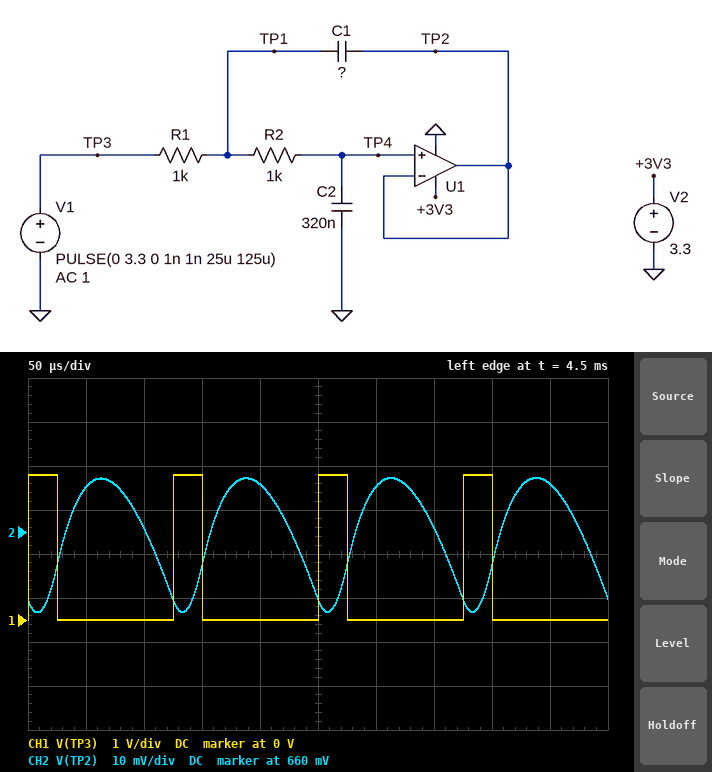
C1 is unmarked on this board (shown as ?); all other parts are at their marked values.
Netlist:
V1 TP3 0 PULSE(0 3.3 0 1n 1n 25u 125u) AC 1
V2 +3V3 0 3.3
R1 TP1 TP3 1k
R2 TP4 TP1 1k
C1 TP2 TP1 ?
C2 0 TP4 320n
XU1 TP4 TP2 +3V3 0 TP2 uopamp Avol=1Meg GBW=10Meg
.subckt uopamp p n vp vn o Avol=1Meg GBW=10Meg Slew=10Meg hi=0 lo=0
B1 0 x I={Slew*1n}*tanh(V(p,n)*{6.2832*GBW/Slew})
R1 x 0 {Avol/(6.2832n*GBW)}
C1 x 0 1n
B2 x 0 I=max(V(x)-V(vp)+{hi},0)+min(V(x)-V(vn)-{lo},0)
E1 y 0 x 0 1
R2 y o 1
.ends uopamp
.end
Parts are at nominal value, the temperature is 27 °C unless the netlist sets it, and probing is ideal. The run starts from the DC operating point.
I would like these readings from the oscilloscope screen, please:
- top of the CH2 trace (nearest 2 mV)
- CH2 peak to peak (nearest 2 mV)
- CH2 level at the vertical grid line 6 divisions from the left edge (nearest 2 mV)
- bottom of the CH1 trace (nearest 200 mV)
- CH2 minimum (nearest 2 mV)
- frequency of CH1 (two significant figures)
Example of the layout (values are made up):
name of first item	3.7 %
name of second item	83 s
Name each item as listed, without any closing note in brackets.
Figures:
top of the CH2 trace	672 mV
CH2 peak to peak	30 mV
CH2 level at the vertical grid line 6 divisions from the left edge	670 mV
bottom of the CH1 trace	0 V
CH2 minimum	642 mV
frequency of CH1	8.0 kHz
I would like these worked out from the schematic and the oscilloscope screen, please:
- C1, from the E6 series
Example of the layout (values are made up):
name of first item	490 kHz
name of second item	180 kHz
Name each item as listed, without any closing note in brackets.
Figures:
C1, from the E6 series	100 nF
